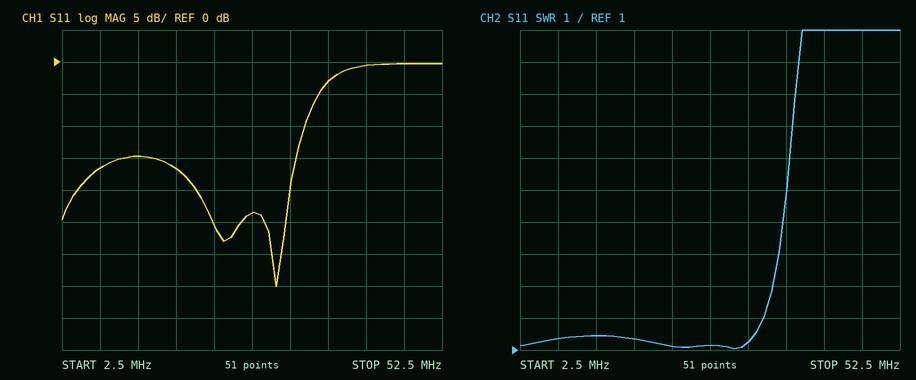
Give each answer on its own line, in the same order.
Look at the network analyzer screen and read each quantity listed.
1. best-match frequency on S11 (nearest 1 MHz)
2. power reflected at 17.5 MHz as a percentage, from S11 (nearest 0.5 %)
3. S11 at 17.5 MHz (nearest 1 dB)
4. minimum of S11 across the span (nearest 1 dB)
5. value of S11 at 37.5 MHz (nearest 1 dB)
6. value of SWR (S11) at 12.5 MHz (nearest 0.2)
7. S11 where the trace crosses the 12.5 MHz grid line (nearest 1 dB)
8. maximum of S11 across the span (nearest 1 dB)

31 MHz
2.0 %
-17 dB
-35 dB
-3 dB
1.4
-15 dB
0 dB
